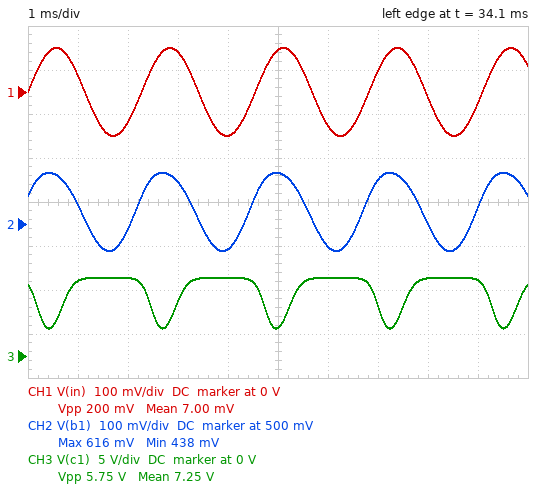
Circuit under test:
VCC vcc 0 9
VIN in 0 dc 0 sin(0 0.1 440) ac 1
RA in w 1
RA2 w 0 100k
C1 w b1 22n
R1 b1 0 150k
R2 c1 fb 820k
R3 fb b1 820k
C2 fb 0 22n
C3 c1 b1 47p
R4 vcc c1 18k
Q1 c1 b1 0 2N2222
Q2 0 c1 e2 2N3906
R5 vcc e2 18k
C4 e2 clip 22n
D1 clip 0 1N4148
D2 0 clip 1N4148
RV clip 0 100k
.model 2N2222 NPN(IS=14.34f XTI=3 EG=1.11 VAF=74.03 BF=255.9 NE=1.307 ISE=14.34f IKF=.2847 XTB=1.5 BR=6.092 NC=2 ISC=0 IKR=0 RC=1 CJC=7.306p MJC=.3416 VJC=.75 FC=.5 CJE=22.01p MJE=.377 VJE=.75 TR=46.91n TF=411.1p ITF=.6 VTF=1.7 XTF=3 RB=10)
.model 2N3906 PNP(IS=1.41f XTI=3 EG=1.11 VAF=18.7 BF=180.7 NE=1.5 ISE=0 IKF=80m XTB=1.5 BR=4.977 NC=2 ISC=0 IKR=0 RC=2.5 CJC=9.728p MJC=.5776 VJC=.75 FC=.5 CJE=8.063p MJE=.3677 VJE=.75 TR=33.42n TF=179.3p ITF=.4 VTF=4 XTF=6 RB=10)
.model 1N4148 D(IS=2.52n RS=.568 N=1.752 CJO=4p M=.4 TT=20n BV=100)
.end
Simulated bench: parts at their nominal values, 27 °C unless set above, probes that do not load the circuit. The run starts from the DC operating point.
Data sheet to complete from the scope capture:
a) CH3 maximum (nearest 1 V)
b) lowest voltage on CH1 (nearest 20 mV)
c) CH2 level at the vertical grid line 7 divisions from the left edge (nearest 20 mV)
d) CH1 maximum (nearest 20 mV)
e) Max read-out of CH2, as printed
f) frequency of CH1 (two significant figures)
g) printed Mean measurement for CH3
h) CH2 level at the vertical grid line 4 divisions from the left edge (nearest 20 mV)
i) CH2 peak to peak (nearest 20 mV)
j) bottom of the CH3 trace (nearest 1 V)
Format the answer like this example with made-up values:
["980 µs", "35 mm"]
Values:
["9 V", "-100 mV", "600 mV", "100 mV", "616 mV", "440 Hz", "7.25 V", "440 mV", "180 mV", "3 V"]
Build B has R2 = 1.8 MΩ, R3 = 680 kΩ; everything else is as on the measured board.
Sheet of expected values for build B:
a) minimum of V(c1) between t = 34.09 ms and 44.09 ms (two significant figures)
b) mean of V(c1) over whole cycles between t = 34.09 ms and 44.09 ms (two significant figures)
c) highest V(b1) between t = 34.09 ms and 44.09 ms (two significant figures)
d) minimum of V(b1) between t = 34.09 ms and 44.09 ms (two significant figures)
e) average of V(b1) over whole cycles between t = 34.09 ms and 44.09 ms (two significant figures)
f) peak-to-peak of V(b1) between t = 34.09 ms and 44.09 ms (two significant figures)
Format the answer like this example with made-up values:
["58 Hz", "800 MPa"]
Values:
["7.8 V", "8.7 V", "570 mV", "380 mV", "480 mV", "190 mV"]
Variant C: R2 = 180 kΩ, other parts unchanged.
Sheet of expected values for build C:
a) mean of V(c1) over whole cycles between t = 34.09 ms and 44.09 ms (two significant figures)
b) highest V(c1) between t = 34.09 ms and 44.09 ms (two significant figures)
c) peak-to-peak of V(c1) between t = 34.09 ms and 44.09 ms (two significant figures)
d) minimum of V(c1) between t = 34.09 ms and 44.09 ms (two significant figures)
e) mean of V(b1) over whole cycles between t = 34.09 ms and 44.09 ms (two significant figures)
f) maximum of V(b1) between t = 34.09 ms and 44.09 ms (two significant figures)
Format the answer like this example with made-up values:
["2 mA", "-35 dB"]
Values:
["5.8 V", "8.6 V", "8.5 V", "91 mV", "560 mV", "630 mV"]
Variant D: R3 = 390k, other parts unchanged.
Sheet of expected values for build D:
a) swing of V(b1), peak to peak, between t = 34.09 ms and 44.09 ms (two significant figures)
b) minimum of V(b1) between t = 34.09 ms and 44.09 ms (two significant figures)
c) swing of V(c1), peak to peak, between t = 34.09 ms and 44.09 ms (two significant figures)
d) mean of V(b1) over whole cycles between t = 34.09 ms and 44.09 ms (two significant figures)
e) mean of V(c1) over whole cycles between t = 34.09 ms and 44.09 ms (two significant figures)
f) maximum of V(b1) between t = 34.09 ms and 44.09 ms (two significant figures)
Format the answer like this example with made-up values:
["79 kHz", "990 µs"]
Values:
["160 mV", "460 mV", "8.7 V", "550 mV", "6.3 V", "630 mV"]
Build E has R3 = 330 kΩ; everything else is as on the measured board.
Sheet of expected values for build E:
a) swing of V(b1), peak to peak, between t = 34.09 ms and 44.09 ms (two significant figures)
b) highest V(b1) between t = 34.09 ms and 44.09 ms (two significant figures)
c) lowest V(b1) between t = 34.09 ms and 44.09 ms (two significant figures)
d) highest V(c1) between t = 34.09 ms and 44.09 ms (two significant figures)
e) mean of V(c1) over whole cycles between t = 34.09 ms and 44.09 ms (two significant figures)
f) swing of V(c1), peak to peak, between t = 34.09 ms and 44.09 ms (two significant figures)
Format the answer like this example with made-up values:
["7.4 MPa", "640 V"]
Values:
["160 mV", "630 mV", "470 mV", "8.8 V", "6.2 V", "8.7 V"]
